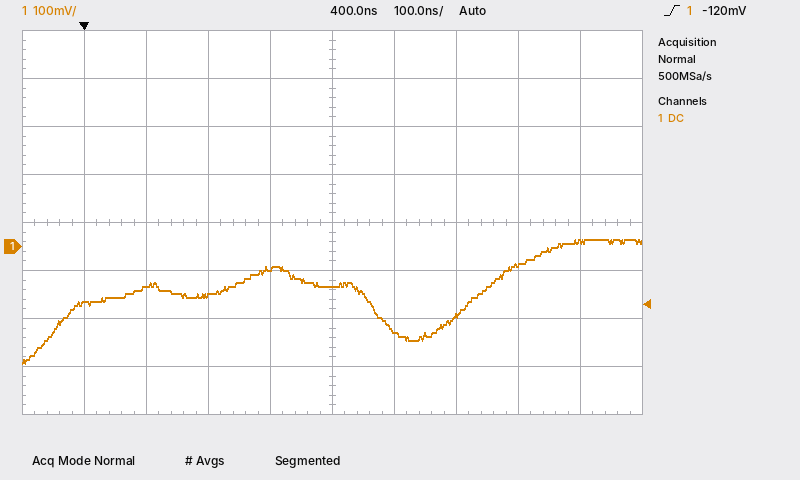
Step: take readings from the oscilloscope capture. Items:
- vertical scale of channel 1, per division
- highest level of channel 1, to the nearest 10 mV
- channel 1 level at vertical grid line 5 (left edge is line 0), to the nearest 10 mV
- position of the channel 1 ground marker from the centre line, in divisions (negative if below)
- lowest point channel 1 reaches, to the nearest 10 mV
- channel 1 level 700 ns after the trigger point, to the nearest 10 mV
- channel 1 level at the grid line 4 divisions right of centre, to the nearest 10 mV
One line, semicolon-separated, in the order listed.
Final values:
100 mV; 10 mV; -80 mV; -0.5 div; -240 mV; -40 mV; 10 mV
